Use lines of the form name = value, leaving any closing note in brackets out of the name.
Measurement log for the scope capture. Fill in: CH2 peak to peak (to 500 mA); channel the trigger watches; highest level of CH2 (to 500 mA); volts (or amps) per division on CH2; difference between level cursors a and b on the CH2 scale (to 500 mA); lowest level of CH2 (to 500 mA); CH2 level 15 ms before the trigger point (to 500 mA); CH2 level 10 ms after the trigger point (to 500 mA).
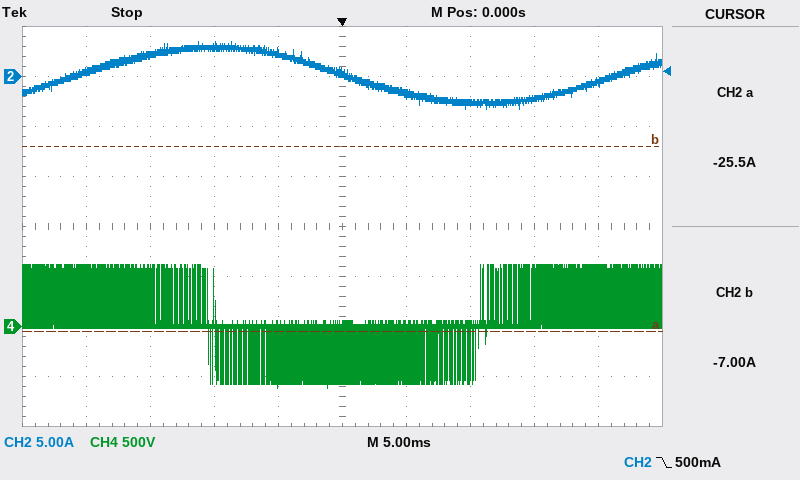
CH2 peak to peak = 7.0 A
channel the trigger watches = CH2
highest level of CH2 = 3.5 A
volts (or amps) per division on CH2 = 5 A
difference between level cursors a and b on the CH2 scale = 18.5 A
lowest level of CH2 = -3.5 A
CH2 level 15 ms before the trigger point = 2.0 A
CH2 level 10 ms after the trigger point = -2.5 A
